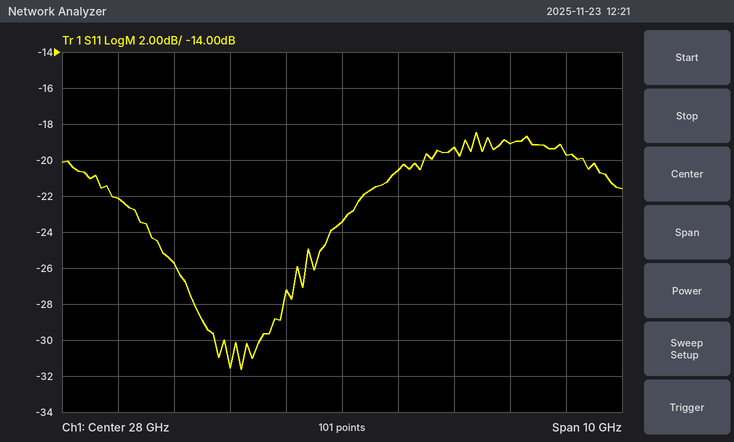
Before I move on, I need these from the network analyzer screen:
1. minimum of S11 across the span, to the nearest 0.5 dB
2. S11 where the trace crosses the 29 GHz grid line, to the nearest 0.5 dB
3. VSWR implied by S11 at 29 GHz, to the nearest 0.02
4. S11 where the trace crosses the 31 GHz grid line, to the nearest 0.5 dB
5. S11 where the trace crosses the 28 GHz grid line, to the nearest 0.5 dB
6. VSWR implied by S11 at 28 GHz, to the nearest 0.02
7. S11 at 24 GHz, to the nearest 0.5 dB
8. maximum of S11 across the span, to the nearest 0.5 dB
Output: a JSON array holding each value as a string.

["-31.5 dB", "-20.5 dB", "1.20", "-19.0 dB", "-23.5 dB", "1.14", "-22.0 dB", "-18.5 dB"]
